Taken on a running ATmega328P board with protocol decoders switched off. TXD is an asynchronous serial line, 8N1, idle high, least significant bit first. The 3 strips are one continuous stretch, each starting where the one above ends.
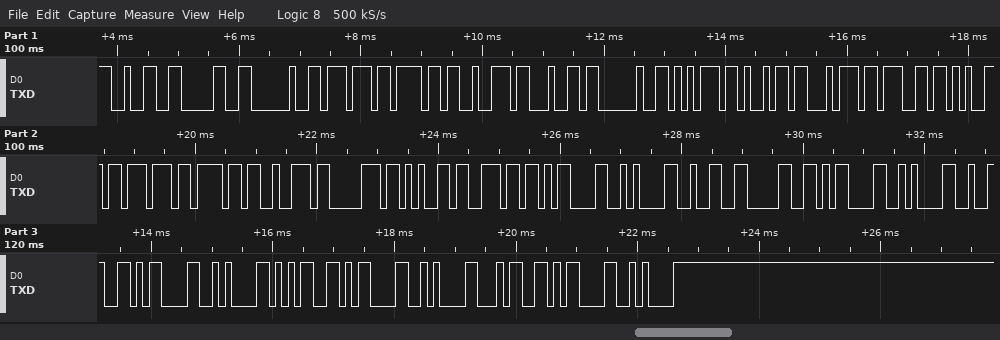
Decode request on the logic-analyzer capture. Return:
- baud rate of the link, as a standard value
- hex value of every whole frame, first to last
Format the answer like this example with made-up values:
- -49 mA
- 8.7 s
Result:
- 9600 baud
- 0x32 0x30 0x20 0x77 0x6F 0x72 0x64 0x20 0x75 0x69 0x74 0x67 0x65 0x77 0x6F 0x72 0x70 0x65 0x6E 0x0D 0x0A 0x32 0x30 0x0D 0x0A 0x32 0x0D 0x0A 0x35 0x0D 0x0A 0x34 0x0D 0x0A
